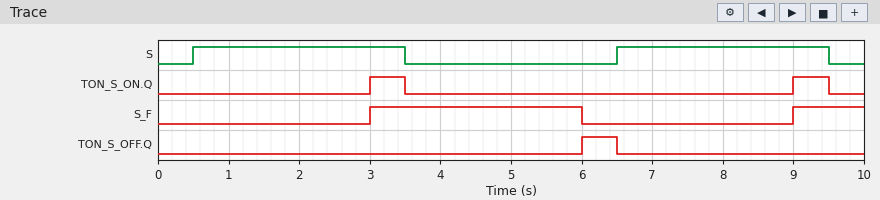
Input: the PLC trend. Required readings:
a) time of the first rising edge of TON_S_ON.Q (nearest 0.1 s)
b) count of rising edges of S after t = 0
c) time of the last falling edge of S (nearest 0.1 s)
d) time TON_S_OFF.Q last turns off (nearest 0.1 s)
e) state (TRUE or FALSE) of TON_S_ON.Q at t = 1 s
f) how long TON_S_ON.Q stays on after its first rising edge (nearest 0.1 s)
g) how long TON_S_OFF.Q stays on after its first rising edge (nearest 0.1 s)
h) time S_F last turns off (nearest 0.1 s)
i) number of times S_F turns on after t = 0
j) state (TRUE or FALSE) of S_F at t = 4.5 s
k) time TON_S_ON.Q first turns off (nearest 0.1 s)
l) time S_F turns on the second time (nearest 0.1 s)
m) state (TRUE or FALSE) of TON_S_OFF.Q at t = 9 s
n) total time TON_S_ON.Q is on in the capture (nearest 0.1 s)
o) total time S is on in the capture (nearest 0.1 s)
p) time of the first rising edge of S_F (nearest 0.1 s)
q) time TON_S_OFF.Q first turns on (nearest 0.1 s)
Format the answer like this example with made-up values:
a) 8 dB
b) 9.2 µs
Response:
a) 3.0 s
b) 2
c) 9.5 s
d) 6.5 s
e) FALSE
f) 0.5 s
g) 0.5 s
h) 6.0 s
i) 2
j) TRUE
k) 3.5 s
l) 9.0 s
m) FALSE
n) 1.0 s
o) 6.0 s
p) 3.0 s
q) 6.0 s
